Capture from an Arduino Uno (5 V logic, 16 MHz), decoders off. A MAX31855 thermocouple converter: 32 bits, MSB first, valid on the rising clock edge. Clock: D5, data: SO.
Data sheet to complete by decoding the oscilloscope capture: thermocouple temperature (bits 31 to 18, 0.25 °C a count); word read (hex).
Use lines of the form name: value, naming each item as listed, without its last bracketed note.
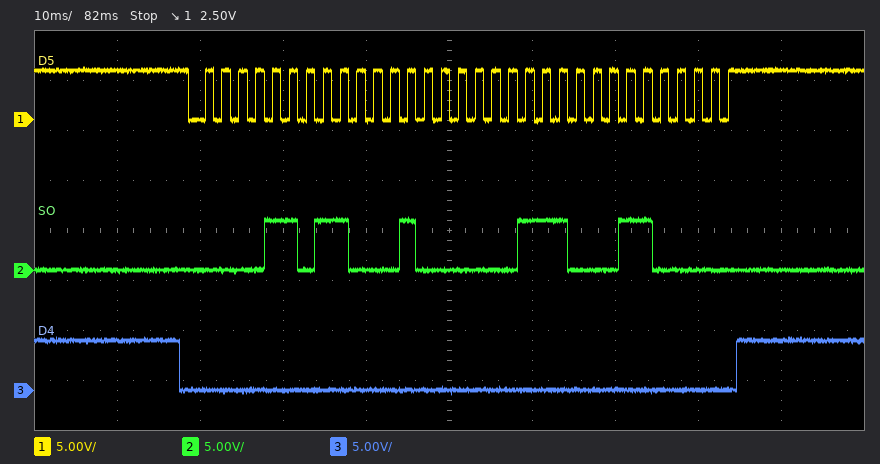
thermocouple temperature: 216.50 °C
word read: 0x0D881C60
